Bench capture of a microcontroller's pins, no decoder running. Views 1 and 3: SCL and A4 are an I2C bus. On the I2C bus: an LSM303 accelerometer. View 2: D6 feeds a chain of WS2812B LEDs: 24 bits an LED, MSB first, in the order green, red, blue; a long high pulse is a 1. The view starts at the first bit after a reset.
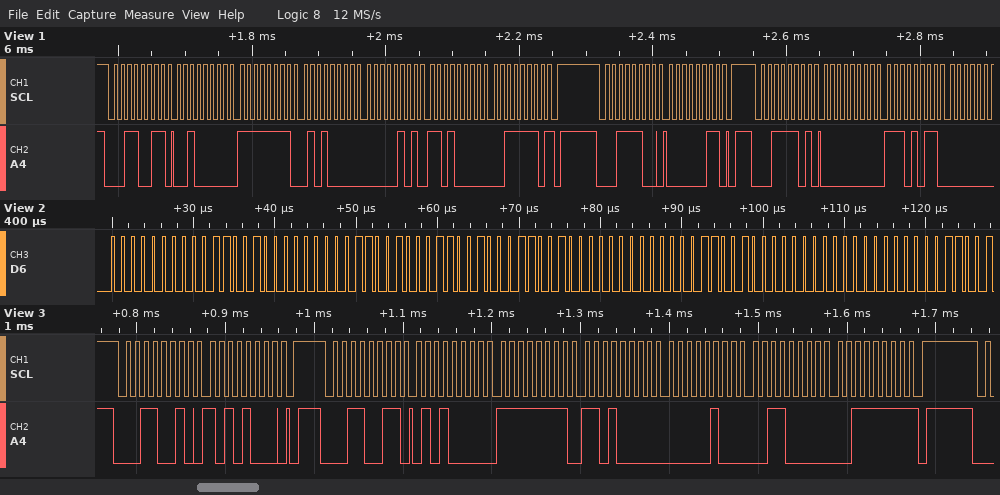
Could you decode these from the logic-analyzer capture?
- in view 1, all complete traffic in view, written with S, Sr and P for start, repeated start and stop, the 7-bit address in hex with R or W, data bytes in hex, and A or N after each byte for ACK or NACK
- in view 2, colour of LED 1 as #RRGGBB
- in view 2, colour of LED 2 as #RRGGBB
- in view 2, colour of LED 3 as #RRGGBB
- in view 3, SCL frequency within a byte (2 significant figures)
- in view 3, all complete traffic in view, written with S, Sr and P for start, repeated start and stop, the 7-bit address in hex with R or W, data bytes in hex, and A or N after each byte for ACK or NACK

S 19R A 20 A FF A 50 A 05 A D0 A 3E N P S 1EW A 03 A P S 1ER A 00 A EB A
#320000
#C8C8C8
#320000
100 kHz
S 19W A A8 A P S 19R A 50 A FF A D0 A 04 A 30 A 3F N P
